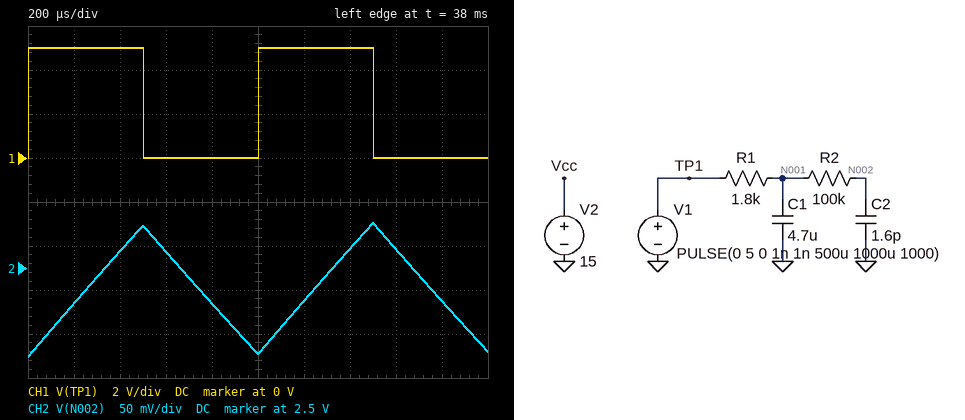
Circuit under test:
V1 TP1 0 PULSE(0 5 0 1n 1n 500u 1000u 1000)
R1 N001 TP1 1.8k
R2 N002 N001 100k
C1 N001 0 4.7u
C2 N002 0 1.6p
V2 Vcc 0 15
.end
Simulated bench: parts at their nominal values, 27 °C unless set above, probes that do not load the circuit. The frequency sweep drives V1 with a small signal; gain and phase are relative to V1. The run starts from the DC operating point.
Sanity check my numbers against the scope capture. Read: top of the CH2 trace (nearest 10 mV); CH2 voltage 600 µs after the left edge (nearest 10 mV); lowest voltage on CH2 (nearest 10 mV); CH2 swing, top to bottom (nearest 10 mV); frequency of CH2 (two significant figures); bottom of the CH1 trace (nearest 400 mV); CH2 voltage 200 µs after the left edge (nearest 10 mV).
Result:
2.55 V
2.52 V
2.40 V
150 mV
1.0 kHz
0 V
2.46 V
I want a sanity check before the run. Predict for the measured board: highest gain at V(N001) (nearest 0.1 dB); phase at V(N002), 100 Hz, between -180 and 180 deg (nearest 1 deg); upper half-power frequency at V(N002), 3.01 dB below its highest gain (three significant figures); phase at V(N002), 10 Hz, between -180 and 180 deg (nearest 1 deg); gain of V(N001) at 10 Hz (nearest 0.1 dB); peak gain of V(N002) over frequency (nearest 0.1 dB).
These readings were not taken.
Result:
0 dB
-79 deg
18.8 Hz
-28 deg
-1.1 dB
0 dB
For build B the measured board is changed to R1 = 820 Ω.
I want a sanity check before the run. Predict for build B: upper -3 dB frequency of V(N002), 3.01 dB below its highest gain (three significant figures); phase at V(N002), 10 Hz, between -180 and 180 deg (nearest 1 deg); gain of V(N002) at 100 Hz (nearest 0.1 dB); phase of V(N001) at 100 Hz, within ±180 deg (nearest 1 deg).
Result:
41.3 Hz
-14 deg
-8.4 dB
-68 deg
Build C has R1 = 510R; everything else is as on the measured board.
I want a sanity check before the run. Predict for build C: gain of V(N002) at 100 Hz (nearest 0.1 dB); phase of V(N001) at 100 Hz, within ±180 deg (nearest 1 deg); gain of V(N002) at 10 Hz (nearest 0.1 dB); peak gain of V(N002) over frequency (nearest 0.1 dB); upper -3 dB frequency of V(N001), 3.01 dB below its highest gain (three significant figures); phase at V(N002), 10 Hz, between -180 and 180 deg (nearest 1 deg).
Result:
-5.1 dB
-56 deg
-0.1 dB
0 dB
66.4 Hz
-9 deg
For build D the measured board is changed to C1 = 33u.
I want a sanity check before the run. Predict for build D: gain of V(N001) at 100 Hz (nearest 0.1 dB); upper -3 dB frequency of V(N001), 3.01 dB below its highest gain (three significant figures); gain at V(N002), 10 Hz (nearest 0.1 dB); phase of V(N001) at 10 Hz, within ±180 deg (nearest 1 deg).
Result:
-31.4 dB
2.68 Hz
-11.7 dB
-75 deg
